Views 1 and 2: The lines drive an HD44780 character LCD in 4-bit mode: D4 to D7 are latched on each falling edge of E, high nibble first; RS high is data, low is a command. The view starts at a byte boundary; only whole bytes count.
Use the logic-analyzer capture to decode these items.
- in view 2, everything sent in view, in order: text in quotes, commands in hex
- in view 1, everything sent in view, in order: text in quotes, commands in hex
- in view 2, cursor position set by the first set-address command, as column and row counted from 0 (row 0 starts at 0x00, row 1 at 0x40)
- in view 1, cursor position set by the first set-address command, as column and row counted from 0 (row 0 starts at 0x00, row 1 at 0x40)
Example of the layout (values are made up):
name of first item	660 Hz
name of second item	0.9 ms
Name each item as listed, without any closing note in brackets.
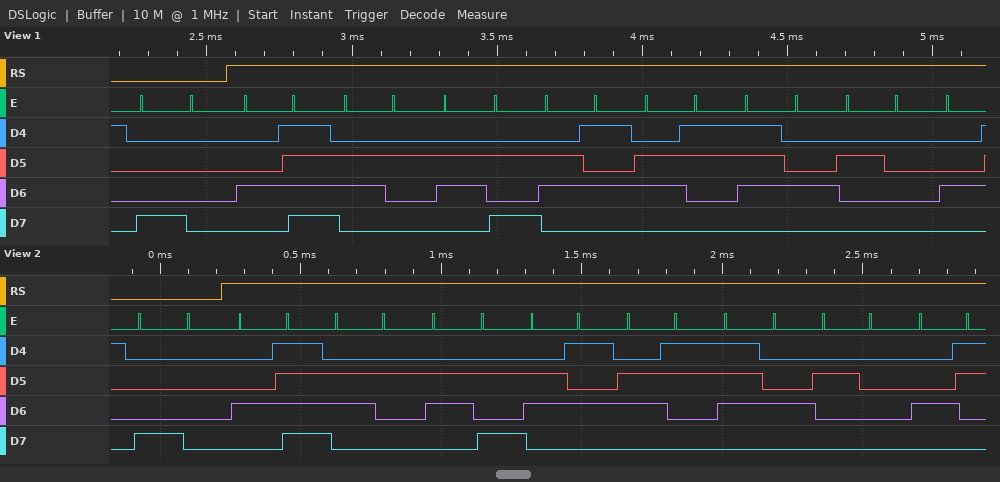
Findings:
in view 2, everything sent in view, in order: text in quotes, commands in hex	0x80 "Object C"
in view 1, everything sent in view, in order: text in quotes, commands in hex	0x80 "Object "
in view 2, cursor position set by the first set-address command, as column and row counted from 0	column 0, row 0
in view 1, cursor position set by the first set-address command, as column and row counted from 0	column 0, row 0
